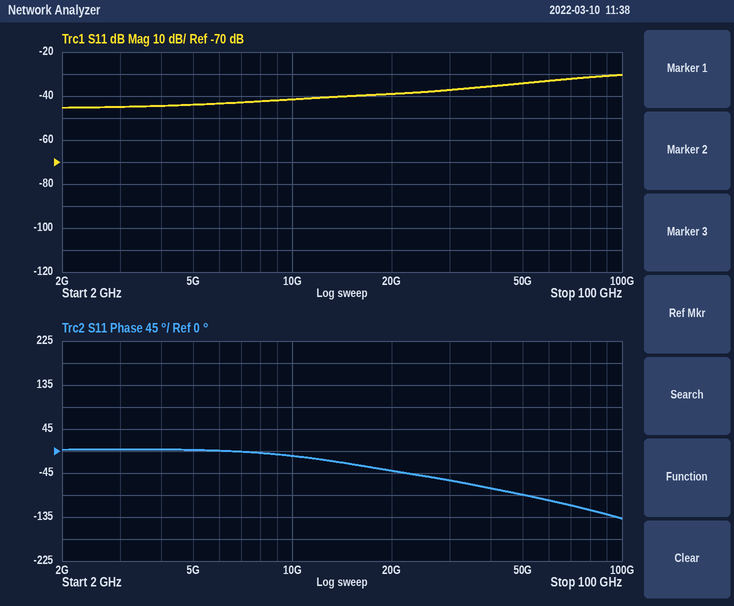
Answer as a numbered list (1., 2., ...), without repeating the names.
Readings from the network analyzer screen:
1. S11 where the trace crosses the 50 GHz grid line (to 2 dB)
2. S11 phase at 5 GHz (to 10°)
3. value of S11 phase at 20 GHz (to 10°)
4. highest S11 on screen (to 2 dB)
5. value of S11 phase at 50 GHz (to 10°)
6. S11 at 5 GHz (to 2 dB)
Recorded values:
1. -34 dB
2. 0°
3. -40°
4. -30 dB
5. -90°
6. -44 dB
